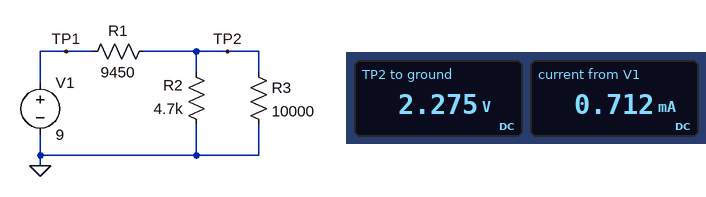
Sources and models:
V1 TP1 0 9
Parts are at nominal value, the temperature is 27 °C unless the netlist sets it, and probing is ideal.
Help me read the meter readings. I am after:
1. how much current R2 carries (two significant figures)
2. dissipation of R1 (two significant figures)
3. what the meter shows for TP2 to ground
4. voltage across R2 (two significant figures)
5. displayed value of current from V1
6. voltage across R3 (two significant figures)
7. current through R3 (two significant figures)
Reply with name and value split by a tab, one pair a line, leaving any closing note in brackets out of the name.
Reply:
how much current R2 carries	480 µA
dissipation of R1	4.8 mW
what the meter shows for TP2 to ground	2.275 V
voltage across R2	2.3 V
displayed value of current from V1	0.712 mA
voltage across R3	2.3 V
current through R3	230 µA
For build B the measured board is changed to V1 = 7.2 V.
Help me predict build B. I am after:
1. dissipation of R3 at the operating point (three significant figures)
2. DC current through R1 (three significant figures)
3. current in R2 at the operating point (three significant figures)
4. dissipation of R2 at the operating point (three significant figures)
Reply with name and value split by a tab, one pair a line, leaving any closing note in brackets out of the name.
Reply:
dissipation of R3 at the operating point	331 µW
DC current through R1	569 µA
current in R2 at the operating point	387 µA
dissipation of R2 at the operating point	705 µW
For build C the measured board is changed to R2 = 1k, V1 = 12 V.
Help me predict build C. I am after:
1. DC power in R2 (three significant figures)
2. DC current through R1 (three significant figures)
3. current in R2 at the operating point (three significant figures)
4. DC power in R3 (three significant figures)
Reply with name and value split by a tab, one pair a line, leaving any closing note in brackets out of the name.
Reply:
DC power in R2	1.11 mW
DC current through R1	1.16 mA
current in R2 at the operating point	1.05 mA
DC power in R3	111 µW
